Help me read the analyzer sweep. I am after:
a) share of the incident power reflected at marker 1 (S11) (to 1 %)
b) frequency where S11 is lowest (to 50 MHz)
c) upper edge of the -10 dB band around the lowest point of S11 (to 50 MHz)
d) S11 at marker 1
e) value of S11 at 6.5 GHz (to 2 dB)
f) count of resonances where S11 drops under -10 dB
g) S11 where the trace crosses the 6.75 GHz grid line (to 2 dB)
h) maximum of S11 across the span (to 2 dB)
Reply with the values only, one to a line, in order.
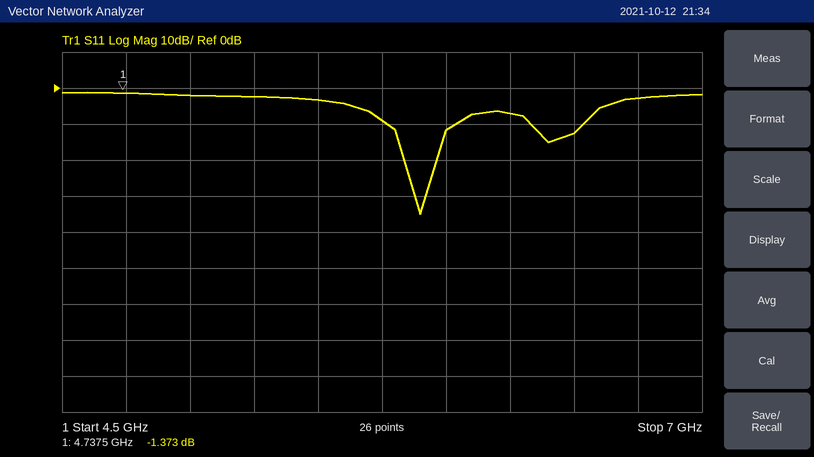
73 %
5.90 GHz
6.05 GHz
-1.373 dB
-12 dB
2
-2 dB
-2 dB
